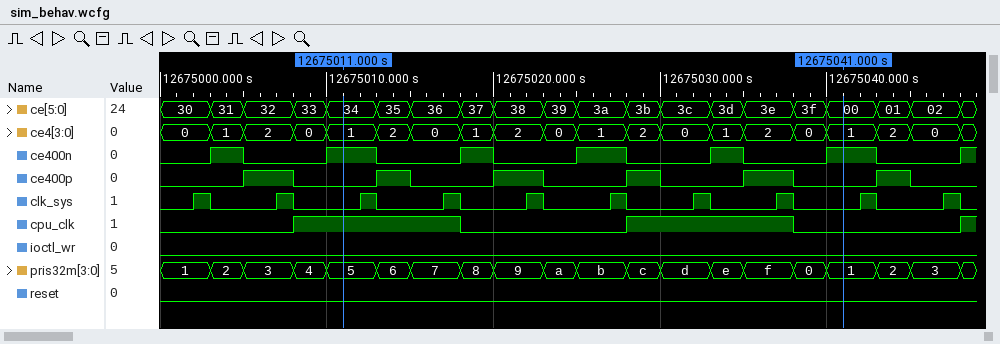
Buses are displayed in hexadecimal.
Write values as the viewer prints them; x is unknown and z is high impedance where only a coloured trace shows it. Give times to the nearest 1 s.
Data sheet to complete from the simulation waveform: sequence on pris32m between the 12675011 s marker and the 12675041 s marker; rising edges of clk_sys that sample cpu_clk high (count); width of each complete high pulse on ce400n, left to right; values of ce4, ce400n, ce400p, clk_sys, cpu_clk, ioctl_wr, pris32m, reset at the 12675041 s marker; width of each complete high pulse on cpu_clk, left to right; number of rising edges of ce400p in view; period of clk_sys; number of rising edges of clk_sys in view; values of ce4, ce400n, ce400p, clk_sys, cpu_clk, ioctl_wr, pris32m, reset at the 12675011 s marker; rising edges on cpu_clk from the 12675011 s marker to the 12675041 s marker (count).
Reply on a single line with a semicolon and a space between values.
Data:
5, 6, 7, 8, 9, a, b, c, d, e, f, 0, 1; 4; 2 s, 3 s, 2 s, 3 s, 2 s, 3 s; ce4=1, ce400n=1, ce400p=0, clk_sys=0, cpu_clk=0, ioctl_wr=0, pris32m=1, reset=0; 10 s, 10 s; 6; 5 s; 10; ce4=1, ce400n=1, ce400p=0, clk_sys=0, cpu_clk=1, ioctl_wr=0, pris32m=5, reset=0; 1
